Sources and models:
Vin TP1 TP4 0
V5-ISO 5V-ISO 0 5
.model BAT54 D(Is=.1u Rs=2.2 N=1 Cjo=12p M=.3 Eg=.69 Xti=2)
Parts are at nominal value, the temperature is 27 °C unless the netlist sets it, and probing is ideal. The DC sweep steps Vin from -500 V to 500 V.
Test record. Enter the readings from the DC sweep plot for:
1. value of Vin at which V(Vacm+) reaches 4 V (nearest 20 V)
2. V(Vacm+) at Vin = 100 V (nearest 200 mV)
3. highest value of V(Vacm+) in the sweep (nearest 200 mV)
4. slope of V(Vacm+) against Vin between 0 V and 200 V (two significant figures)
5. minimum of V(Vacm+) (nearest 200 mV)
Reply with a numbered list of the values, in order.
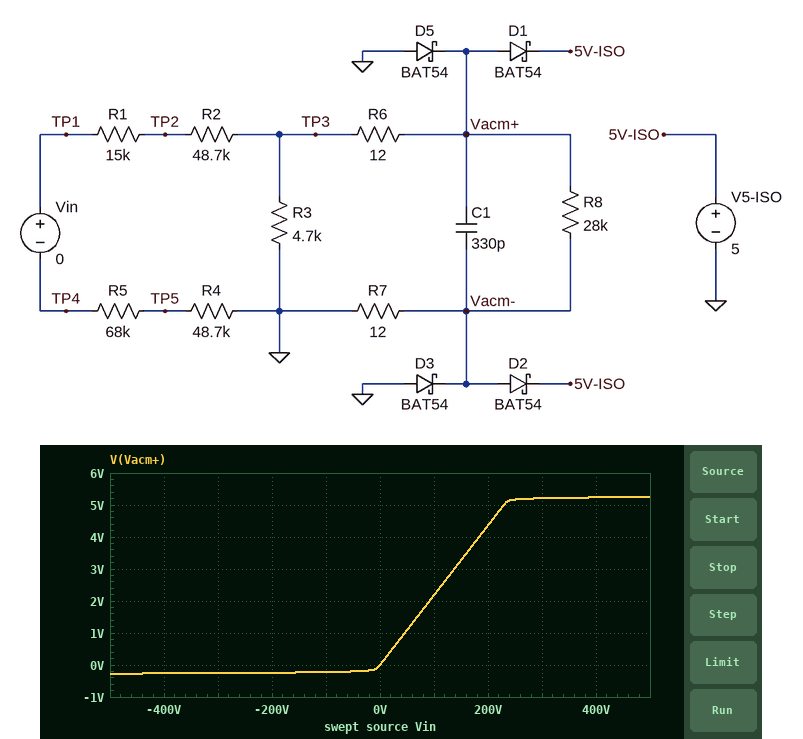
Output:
1. 180 V
2. 2.2 V
3. 5.2 V
4. 0.022 V/V
5. -200 mV
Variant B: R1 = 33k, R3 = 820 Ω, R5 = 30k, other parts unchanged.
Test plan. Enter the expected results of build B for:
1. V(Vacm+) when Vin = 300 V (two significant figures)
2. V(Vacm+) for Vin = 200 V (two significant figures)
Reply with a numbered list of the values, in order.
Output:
1. 1.5 V
2. 990 mV
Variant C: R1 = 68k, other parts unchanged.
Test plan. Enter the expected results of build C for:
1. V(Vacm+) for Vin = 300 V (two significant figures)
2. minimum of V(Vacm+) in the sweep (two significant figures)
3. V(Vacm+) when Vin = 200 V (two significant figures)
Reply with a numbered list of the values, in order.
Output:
1. 5.1 V
2. -260 mV
3. 3.4 V
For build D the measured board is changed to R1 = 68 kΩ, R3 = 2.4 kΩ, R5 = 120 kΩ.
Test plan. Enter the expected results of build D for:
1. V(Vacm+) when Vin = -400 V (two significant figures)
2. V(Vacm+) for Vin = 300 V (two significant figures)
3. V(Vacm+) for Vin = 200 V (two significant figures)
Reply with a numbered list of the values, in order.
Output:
1. -250 mV
2. 2.3 V
3. 1.5 V
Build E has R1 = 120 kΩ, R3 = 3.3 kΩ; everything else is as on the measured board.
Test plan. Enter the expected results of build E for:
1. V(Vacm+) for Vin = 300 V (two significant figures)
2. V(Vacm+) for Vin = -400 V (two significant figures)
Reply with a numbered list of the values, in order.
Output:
1. 3.1 V
2. -250 mV
